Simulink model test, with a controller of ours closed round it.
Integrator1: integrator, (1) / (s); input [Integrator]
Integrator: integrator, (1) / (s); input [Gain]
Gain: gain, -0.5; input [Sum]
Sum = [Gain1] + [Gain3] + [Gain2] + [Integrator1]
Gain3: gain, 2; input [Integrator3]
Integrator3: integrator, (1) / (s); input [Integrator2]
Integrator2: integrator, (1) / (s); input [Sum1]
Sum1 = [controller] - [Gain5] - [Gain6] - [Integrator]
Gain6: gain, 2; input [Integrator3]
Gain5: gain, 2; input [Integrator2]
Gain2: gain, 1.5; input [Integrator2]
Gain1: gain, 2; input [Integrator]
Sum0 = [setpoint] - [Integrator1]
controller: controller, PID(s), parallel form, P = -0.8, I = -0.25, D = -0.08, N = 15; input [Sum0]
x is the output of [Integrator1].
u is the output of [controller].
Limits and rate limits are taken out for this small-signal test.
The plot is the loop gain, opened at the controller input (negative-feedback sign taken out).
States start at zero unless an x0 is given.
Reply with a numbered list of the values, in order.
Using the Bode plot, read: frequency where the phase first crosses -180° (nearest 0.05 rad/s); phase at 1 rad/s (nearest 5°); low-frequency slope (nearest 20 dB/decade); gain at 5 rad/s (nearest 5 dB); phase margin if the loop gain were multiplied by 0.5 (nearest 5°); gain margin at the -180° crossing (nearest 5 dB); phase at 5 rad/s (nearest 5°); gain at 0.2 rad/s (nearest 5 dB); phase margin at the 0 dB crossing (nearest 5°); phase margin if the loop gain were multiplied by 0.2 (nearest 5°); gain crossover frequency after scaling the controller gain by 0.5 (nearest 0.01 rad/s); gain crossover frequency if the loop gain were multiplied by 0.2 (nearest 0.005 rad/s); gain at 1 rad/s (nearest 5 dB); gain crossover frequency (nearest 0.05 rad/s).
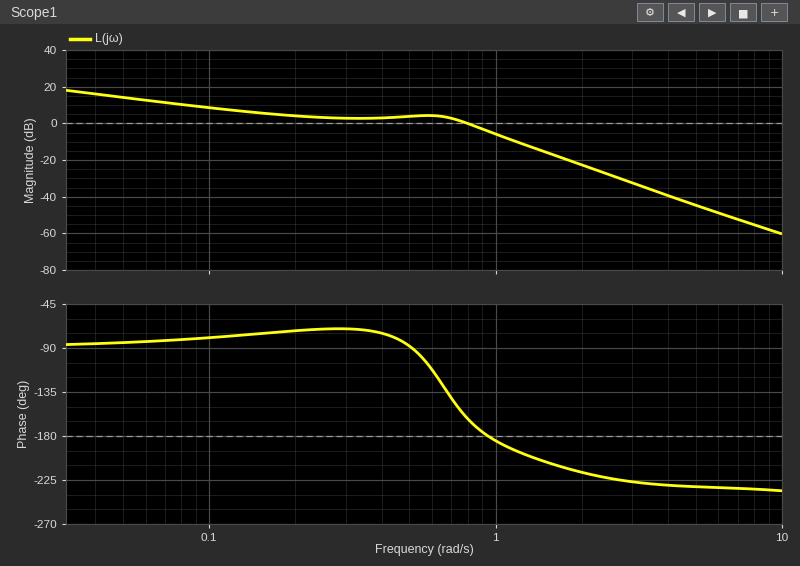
1. 0.95 rad/s
2. -185°
3. -20 dB/decade
4. -45 dB
5. 105°
6. 5 dB
7. -230°
8. 5 dB
9. 20°
10. 95°
11. 0.14 rad/s
12. 0.050 rad/s
13. -5 dB
14. 0.80 rad/s
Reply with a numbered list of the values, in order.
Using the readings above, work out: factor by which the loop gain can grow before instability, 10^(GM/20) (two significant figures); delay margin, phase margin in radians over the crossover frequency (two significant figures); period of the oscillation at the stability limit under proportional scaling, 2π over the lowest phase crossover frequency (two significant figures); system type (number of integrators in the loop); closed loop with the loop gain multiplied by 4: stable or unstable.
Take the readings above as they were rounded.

1. 1.8
2. 0.44 s
3. 6.6 s
4. 1
5. unstable
